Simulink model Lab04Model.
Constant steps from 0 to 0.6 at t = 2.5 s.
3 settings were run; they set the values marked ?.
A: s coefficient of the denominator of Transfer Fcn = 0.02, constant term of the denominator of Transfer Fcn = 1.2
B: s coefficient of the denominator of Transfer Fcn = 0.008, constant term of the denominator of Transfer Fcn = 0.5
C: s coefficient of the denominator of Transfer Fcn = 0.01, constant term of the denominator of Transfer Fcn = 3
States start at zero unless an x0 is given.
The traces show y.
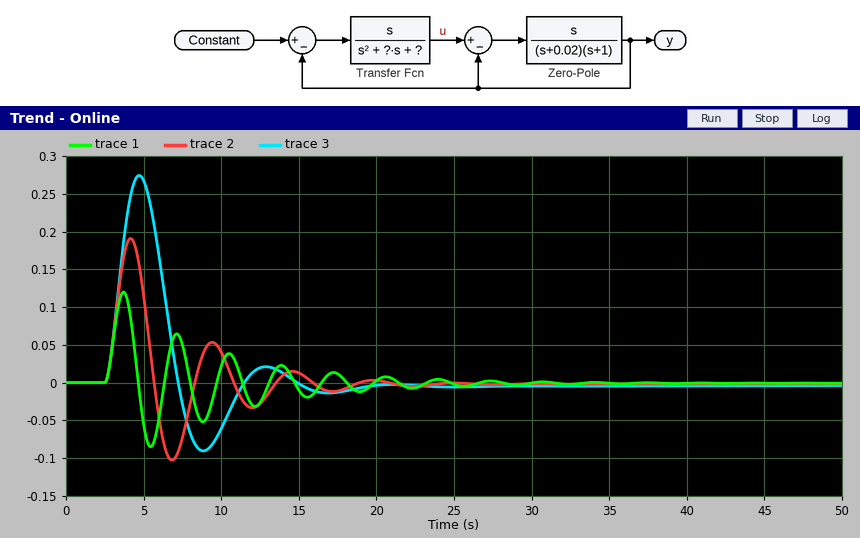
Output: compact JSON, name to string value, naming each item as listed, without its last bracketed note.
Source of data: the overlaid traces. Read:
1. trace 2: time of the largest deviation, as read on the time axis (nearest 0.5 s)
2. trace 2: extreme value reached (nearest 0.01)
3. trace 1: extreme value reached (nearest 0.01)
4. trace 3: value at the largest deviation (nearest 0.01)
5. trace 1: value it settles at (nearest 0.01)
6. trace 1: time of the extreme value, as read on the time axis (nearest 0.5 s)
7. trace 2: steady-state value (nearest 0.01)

{"trace 2: time of the largest deviation, as read on the time axis": "4.0 s", "trace 2: extreme value reached": "0.19", "trace 1: extreme value reached": "0.12", "trace 3: value at the largest deviation": "0.27", "trace 1: value it settles at": "0.00", "trace 1: time of the extreme value, as read on the time axis": "3.5 s", "trace 2: steady-state value": "0.00"}
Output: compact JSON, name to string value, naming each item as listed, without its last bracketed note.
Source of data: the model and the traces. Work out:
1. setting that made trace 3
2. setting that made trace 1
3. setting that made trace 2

{"setting that made trace 3": "B", "setting that made trace 1": "C", "setting that made trace 2": "A"}
